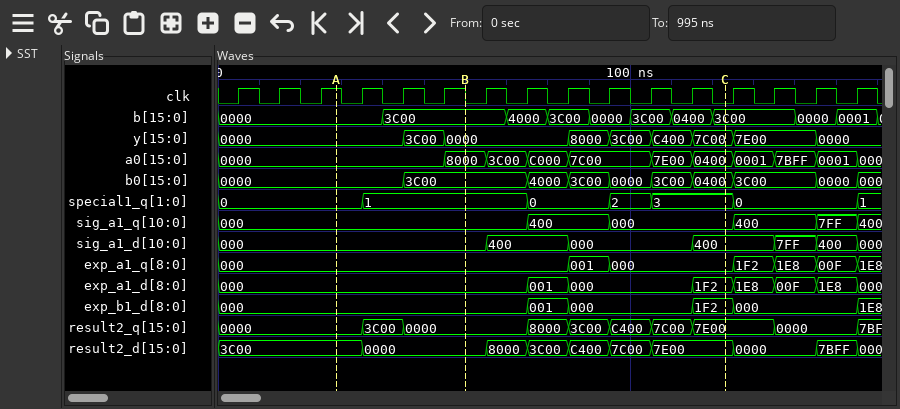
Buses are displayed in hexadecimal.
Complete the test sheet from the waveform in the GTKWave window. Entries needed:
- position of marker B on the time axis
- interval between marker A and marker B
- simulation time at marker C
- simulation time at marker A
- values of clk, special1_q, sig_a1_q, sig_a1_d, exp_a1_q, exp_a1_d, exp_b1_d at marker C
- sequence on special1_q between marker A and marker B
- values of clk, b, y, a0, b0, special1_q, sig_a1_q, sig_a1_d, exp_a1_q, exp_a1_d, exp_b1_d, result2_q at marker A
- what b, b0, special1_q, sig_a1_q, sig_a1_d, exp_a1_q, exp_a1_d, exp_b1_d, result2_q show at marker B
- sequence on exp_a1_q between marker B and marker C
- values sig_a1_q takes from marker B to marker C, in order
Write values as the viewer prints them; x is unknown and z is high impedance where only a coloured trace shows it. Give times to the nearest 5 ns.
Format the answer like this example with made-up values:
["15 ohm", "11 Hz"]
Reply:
["60 ns", "30 ns", "125 ns", "30 ns", "clk=0, special1_q=3, sig_a1_q=000, sig_a1_d=400, exp_a1_q=000, exp_a1_d=1F2, exp_b1_d=1F2", "0, 1", "clk=1, b=0000, y=0000, a0=0000, b0=0000, special1_q=0, sig_a1_q=000, sig_a1_d=000, exp_a1_q=000, exp_a1_d=000, exp_b1_d=000, result2_q=0000", "b=3C00, b0=3C00, special1_q=1, sig_a1_q=000, sig_a1_d=000, exp_a1_q=000, exp_a1_d=000, exp_b1_d=000, result2_q=0000", "000, 001, 000", "000, 400, 000"]
